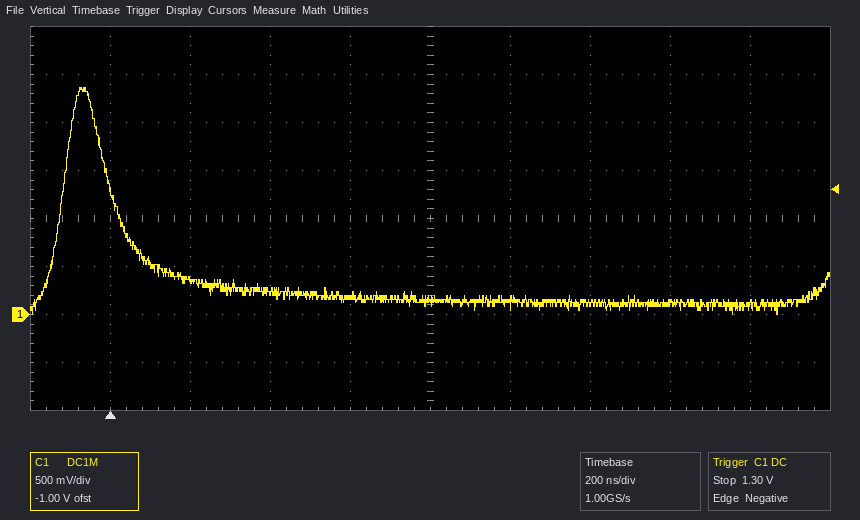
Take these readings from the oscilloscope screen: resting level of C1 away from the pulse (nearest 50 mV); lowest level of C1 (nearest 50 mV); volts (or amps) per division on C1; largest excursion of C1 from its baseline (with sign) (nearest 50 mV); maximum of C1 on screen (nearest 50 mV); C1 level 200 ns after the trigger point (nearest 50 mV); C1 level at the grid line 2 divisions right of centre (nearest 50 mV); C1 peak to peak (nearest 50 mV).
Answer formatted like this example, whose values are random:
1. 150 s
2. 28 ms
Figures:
1. 150 mV
2. 0 mV
3. 500 mV
4. +2.20 V
5. 2.35 V
6. 350 mV
7. 100 mV
8. 2.35 V
